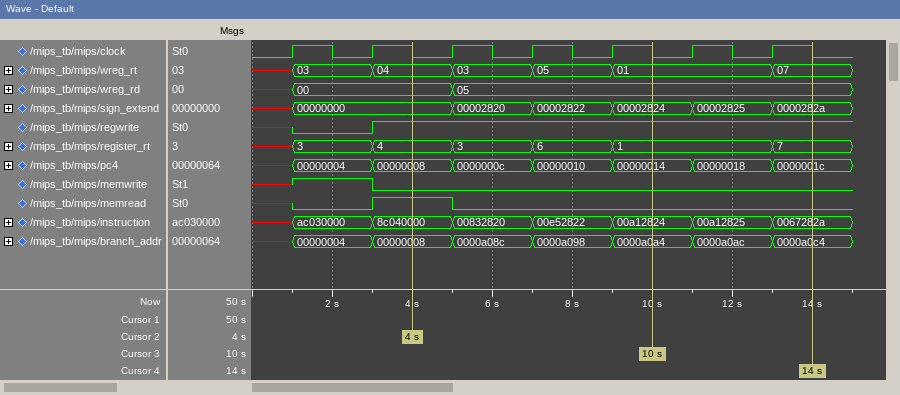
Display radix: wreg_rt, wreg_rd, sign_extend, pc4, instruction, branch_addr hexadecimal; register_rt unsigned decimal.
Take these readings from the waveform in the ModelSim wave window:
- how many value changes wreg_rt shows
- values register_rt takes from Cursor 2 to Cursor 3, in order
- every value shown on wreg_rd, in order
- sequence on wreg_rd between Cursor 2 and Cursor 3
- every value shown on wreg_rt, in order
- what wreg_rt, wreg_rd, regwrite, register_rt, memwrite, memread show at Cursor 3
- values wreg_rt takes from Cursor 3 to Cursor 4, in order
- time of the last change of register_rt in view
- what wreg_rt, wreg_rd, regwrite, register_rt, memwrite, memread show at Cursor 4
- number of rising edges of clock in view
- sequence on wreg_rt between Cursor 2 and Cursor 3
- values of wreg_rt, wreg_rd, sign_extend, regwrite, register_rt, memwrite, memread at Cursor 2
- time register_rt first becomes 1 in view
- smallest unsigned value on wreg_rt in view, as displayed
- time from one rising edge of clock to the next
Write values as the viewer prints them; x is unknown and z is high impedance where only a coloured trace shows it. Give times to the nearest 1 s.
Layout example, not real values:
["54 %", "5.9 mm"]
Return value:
["6", "4, 3, 6, 1", "x, 00, 05", "00, 05", "x, 03, 04, 03, 05, 01, 07", "wreg_rt=01, wreg_rd=05, regwrite=1, register_rt=1, memwrite=0, memread=0", "01, 07", "13 s", "wreg_rt=07, wreg_rd=05, regwrite=1, register_rt=7, memwrite=0, memread=0", "7", "04, 03, 05, 01", "wreg_rt=04, wreg_rd=00, sign_extend=00000000, regwrite=1, register_rt=4, memwrite=0, memread=1", "9 s", "01", "2 s"]
